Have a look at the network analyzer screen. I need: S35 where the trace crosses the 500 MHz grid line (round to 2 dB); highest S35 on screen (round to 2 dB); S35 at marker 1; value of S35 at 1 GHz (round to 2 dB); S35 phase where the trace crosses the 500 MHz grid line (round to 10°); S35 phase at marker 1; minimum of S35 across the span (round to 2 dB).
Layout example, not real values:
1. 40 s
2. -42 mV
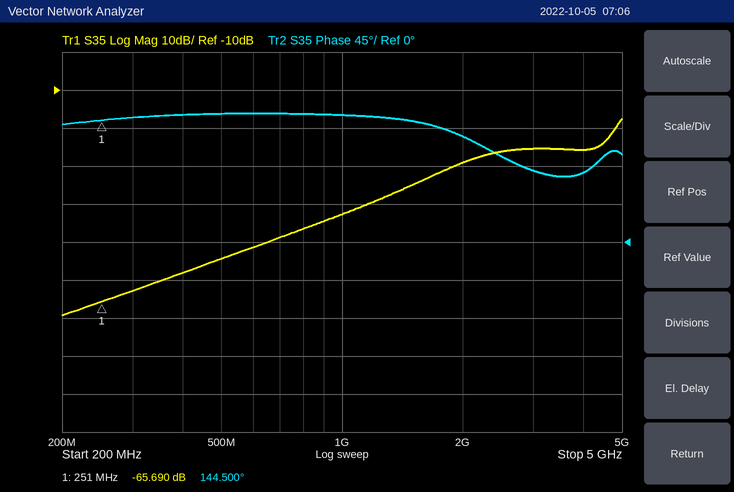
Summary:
1. -54 dB
2. -18 dB
3. -65.690 dB
4. -42 dB
5. 150°
6. 144.500°
7. -70 dB
